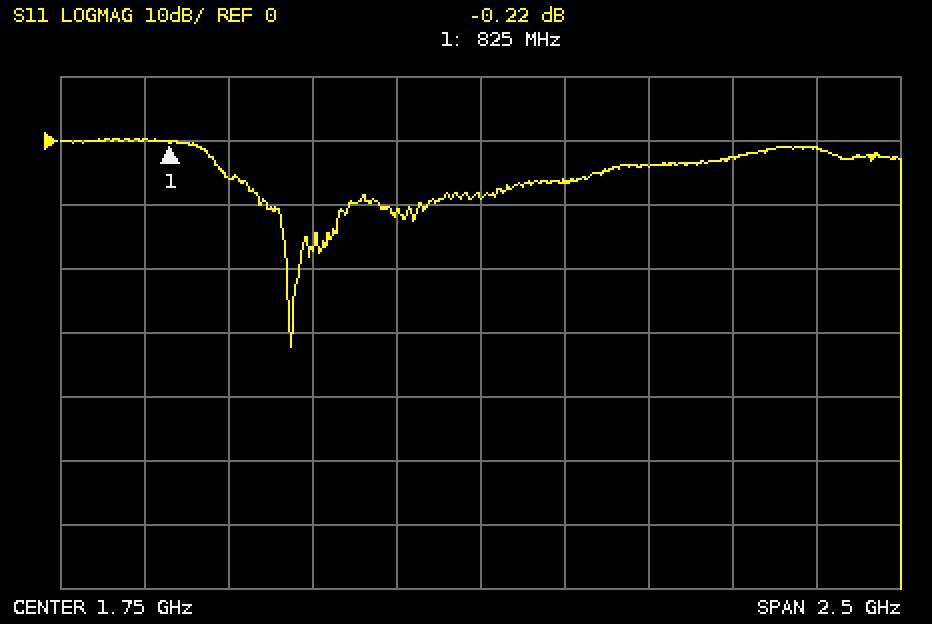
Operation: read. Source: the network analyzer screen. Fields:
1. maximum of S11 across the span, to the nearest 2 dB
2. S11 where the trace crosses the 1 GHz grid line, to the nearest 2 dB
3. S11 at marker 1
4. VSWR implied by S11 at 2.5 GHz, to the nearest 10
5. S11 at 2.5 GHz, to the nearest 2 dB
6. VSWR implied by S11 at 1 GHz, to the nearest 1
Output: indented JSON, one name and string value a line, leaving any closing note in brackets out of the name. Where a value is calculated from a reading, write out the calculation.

{
  "maximum of S11 across the span, to the nearest 2 dB": "0 dB",
  "S11 where the trace crosses the 1 GHz grid line, to the nearest 2 dB": "-6 dB",
  "S11 at marker 1": "-0.22 dB",
  "VSWR implied by S11 at 2.5 GHz, to the nearest 10": "|Γ| = 10^(-2/20) = 0.7943; VSWR = (1 + 0.7943)/(1 − 0.7943) ≈ 8.72, so 10 to the nearest 10",
  "S11 at 2.5 GHz, to the nearest 2 dB": "-2 dB",
  "VSWR implied by S11 at 1 GHz, to the nearest 1": "|Γ| = 10^(-6/20) = 0.5012; VSWR = (1 + 0.5012)/(1 − 0.5012) ≈ 3"
}
